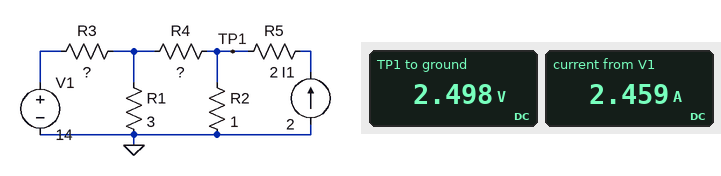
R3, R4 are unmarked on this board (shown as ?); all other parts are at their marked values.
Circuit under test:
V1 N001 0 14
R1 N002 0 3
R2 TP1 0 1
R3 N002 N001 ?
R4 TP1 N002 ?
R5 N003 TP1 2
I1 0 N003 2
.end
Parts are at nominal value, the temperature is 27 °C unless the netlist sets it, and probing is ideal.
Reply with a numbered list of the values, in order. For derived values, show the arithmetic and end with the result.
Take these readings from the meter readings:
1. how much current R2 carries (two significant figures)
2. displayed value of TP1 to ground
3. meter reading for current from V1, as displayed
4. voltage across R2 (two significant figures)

1. (2.498 V) / 1 Ω = 2.5 A
2. 2.498 V
3. 2.459 A
4. 2.498 V = 2.5 V
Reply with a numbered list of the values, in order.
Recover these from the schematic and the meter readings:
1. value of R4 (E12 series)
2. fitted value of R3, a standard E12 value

1. 6.8 Ω
2. 3.3 Ω
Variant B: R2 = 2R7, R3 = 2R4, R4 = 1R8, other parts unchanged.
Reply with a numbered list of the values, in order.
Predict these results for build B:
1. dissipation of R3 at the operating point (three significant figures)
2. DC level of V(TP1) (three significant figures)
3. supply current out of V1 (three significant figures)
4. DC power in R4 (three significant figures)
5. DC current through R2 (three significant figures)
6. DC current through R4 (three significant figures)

1. 19.1 W
2. 6.50 V
3. 2.82 A
4. 299 mW
5. 2.41 A
6. 408 mA
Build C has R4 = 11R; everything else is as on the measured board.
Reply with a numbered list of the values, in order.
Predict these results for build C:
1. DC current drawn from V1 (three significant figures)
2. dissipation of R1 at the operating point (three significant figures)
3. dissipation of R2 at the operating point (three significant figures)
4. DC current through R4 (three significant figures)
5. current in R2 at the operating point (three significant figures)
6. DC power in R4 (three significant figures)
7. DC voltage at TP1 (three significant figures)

1. 2.39 A
2. 12.5 W
3. 5.49 W
4. 344 mA
5. 2.34 A
6. 1.30 W
7. 2.34 V
